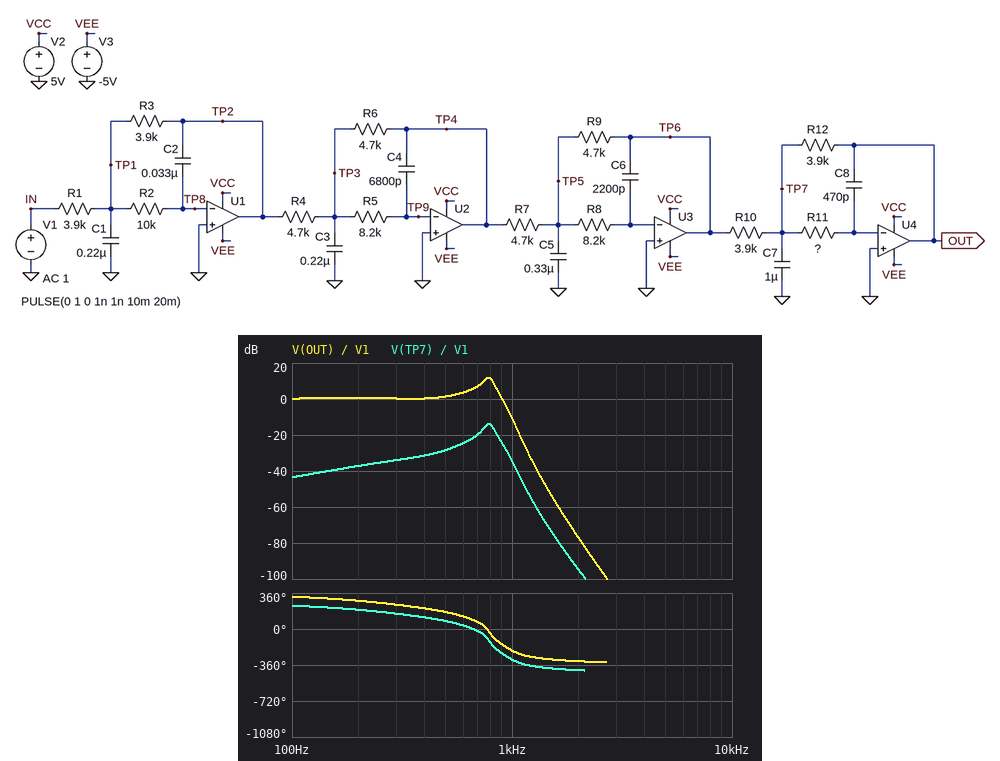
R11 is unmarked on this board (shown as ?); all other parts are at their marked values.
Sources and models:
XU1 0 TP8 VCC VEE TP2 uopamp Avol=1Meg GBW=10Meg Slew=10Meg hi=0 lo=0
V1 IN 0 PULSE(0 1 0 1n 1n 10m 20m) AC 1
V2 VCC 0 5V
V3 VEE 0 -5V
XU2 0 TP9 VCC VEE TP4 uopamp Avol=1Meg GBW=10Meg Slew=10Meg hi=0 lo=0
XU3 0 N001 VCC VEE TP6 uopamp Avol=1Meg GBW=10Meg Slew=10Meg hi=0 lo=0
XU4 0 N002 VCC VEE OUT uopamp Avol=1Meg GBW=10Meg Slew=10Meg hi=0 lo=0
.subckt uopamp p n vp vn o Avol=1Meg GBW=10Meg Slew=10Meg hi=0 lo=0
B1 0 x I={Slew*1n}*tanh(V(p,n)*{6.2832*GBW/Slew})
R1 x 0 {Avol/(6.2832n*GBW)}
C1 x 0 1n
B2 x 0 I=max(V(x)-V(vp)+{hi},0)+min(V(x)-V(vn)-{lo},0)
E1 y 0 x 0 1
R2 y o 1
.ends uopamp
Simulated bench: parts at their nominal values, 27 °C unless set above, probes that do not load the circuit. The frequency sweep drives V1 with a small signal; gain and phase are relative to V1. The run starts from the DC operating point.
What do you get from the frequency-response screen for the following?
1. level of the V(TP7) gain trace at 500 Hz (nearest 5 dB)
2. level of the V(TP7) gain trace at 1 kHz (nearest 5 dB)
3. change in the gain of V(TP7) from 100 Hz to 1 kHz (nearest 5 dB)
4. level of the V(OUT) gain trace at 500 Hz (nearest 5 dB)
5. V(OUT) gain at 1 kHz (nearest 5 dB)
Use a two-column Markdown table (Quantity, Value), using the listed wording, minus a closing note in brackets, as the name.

| Quantity | Value |
|---|---|
| level of the V(TP7) gain trace at 500 Hz | -30 dB |
| level of the V(TP7) gain trace at 1 kHz | -35 dB |
| change in the gain of V(TP7) from 100 Hz to 1 kHz | 10 dB |
| level of the V(OUT) gain trace at 500 Hz | 0 dB |
| V(OUT) gain at 1 kHz | -10 dB |
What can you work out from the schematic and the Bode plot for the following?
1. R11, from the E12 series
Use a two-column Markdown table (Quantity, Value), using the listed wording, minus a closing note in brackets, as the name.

| Quantity | Value |
|---|---|
| R11, from the E12 series | 22 kΩ |
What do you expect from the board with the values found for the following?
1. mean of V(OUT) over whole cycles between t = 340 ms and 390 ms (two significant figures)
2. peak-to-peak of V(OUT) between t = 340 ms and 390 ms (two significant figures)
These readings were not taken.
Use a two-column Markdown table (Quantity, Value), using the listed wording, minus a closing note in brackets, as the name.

| Quantity | Value |
|---|---|
| mean of V(OUT) over whole cycles between t = 340 ms and 390 ms | 500 mV |
| peak-to-peak of V(OUT) between t = 340 ms and 390 ms | 1.7 V |
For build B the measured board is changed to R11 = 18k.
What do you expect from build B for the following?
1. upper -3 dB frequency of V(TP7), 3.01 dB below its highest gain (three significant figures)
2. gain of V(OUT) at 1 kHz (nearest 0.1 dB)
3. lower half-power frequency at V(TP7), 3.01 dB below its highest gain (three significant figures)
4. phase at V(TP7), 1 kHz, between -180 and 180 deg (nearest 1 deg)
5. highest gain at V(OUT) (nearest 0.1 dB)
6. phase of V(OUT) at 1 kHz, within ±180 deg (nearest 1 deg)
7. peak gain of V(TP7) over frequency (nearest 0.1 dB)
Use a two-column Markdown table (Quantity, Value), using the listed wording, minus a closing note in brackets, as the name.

| Quantity | Value |
|---|---|
| upper -3 dB frequency of V(TP7), 3.01 dB below its highest gain | 910 Hz |
| gain of V(OUT) at 1 kHz | -5.1 dB |
| lower half-power frequency at V(TP7), 3.01 dB below its highest gain | 820 Hz |
| phase at V(TP7), 1 kHz, between -180 and 180 deg | 62 deg |
| highest gain at V(OUT) | 10.9 dB |
| phase of V(OUT) at 1 kHz, within ±180 deg | 152 deg |
| peak gain of V(TP7) over frequency | -15.8 dB |
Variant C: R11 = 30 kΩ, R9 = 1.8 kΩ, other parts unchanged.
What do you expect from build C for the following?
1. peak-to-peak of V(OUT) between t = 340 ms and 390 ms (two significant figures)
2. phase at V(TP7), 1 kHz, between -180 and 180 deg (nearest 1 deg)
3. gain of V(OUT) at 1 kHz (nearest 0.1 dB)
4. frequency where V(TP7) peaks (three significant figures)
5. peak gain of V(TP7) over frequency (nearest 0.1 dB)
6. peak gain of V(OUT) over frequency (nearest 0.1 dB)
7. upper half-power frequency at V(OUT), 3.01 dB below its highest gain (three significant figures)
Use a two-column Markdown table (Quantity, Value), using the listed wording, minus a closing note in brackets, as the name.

| Quantity | Value |
|---|---|
| peak-to-peak of V(OUT) between t = 340 ms and 390 ms | 620 mV |
| phase at V(TP7), 1 kHz, between -180 and 180 deg | 143 deg |
| gain of V(OUT) at 1 kHz | -30.4 dB |
| frequency where V(TP7) peaks | 671 Hz |
| peak gain of V(TP7) over frequency | -23.3 dB |
| peak gain of V(OUT) over frequency | 1.2 dB |
| upper half-power frequency at V(OUT), 3.01 dB below its highest gain | 706 Hz |
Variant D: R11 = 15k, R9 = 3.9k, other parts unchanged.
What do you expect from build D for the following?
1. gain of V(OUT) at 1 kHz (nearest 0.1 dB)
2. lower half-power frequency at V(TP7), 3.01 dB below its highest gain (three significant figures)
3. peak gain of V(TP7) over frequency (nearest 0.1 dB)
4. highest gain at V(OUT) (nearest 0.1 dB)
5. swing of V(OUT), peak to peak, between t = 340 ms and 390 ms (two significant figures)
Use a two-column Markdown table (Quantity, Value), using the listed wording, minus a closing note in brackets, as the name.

| Quantity | Value |
|---|---|
| gain of V(OUT) at 1 kHz | 2.2 dB |
| lower half-power frequency at V(TP7), 3.01 dB below its highest gain | 903 Hz |
| peak gain of V(TP7) over frequency | -21.3 dB |
| highest gain at V(OUT) | 6.2 dB |
| swing of V(OUT), peak to peak, between t = 340 ms and 390 ms | 1.2 V |
